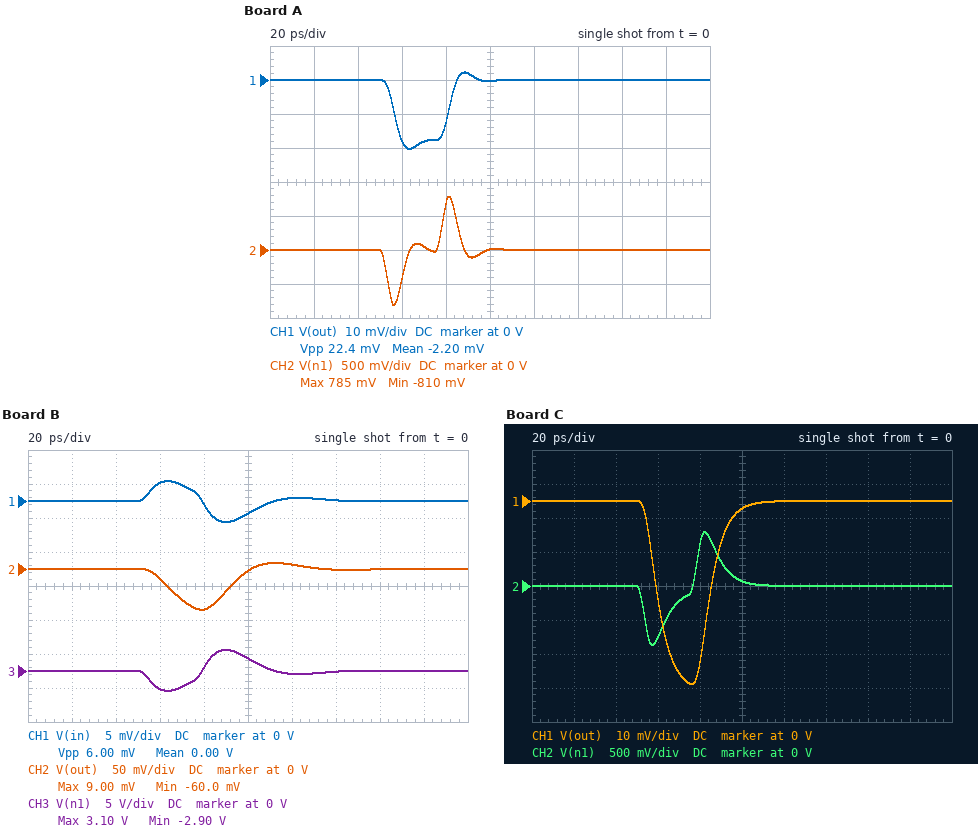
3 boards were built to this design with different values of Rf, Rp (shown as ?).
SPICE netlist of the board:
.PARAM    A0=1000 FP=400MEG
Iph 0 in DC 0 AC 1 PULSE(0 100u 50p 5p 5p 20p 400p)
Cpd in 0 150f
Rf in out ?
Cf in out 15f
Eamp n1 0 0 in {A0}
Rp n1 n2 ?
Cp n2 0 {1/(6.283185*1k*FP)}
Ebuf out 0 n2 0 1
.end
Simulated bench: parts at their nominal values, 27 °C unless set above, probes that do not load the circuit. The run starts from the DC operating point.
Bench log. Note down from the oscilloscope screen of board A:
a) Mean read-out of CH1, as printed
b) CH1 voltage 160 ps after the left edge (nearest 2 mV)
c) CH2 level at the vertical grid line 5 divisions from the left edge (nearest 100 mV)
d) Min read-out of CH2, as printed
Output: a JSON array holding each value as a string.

["-2.20 mV", "0 V", "0 V", "-810 mV"]
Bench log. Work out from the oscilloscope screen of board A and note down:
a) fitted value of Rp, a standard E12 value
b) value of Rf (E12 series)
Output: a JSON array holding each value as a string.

["680 Ω", "180 Ω"]
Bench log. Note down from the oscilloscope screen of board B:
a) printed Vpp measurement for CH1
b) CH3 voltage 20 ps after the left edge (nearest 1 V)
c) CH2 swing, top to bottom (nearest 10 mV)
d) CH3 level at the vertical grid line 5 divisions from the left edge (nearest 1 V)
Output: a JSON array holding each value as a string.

["6.00 mV", "0 V", "70 mV", "2 V"]
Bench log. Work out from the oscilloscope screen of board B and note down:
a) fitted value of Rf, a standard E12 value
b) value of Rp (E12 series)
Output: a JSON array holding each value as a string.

["560 Ω", "2.2 kΩ"]
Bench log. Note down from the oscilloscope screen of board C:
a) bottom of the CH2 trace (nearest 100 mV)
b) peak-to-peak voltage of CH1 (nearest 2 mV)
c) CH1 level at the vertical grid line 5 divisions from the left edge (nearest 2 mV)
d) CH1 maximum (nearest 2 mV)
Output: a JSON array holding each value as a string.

["-900 mV", "54 mV", "-2 mV", "0 V"]
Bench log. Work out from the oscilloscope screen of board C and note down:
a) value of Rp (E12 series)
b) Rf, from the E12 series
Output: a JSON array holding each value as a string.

["470 Ω", "560 Ω"]
